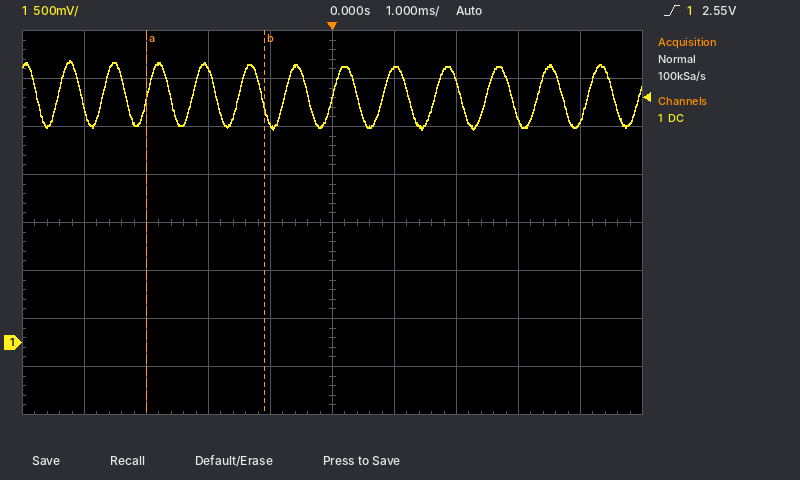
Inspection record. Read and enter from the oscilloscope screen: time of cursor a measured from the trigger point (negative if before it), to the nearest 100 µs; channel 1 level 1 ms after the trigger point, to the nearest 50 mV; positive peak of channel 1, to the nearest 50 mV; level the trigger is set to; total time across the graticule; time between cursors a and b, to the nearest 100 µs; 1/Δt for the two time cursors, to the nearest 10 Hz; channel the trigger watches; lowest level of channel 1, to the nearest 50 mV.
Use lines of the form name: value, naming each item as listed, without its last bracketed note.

time of cursor a measured from the trigger point (negative if before it), to the nearest 100 µs: -3.0 ms
channel 1 level 1 ms after the trigger point, to the nearest 50 mV: 2.85 V
positive peak of channel 1, to the nearest 50 mV: 2.95 V
level the trigger is set to: 2.55 V
total time across the graticule: 10 ms
time between cursors a and b, to the nearest 100 µs: 1.9 ms
1/Δt for the two time cursors, to the nearest 10 Hz: 530 Hz
channel the trigger watches: channel 1
lowest level of channel 1, to the nearest 50 mV: 2.20 V
